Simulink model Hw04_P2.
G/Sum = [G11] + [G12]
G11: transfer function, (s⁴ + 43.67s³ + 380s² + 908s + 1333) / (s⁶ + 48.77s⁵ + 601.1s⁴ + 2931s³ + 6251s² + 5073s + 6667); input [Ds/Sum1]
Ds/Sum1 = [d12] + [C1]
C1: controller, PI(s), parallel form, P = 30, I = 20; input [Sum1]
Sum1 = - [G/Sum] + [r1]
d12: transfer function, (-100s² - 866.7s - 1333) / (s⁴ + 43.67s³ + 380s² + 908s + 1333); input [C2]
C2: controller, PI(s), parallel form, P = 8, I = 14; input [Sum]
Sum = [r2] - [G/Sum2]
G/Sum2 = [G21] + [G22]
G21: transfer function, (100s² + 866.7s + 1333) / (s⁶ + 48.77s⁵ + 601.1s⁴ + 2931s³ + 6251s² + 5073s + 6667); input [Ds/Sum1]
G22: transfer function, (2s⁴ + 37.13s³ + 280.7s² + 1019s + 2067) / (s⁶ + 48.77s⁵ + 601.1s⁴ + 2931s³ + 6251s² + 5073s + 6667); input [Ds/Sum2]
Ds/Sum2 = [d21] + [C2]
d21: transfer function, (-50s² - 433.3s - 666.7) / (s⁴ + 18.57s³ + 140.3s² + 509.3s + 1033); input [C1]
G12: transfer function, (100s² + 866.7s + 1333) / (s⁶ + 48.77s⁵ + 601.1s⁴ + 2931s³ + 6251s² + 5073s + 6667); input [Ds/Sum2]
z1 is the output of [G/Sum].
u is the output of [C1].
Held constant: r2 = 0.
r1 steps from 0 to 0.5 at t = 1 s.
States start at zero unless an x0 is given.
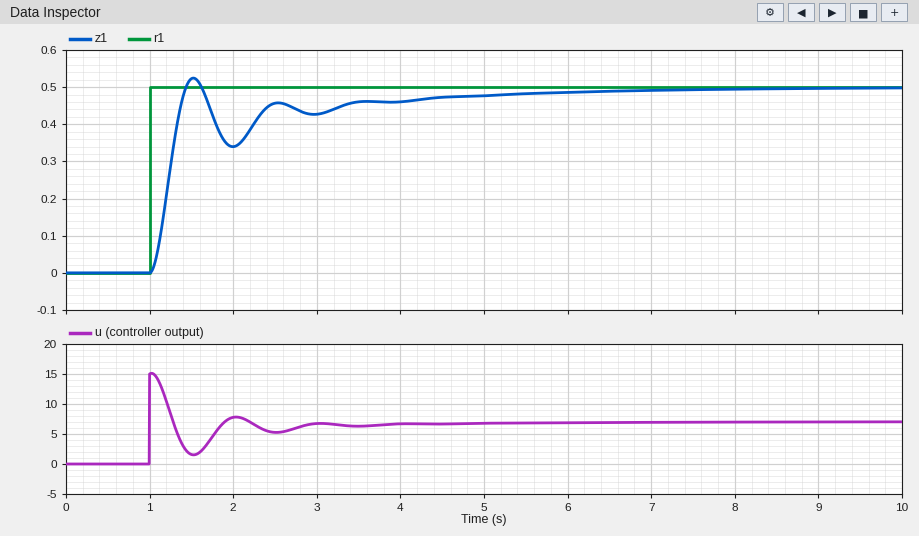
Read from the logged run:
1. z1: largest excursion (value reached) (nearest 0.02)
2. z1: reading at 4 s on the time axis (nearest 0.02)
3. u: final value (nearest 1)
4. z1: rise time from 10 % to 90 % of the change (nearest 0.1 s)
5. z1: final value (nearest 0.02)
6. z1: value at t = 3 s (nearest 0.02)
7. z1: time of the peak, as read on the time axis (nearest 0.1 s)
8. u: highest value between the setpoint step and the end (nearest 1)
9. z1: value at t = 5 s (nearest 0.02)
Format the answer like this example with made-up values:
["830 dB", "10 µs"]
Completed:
["0.52", "0.46", "7", "0.3 s", "0.50", "0.42", "1.5 s", "15", "0.48"]
